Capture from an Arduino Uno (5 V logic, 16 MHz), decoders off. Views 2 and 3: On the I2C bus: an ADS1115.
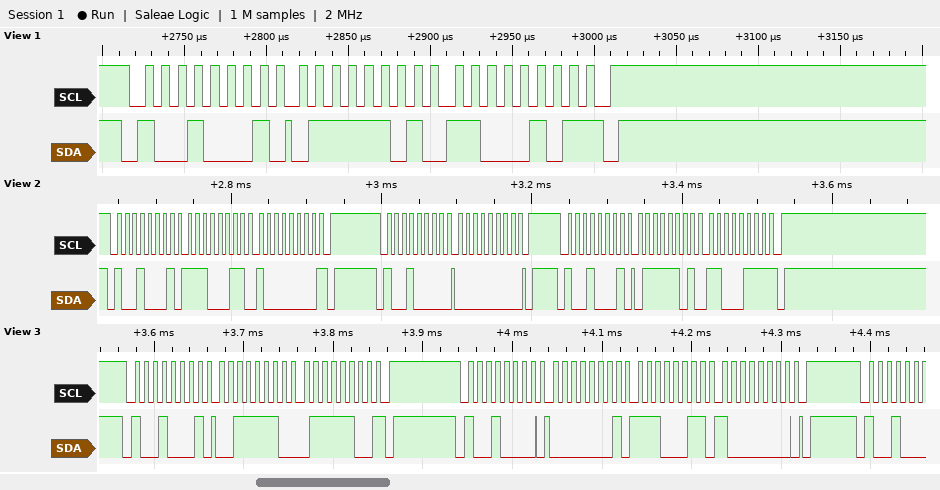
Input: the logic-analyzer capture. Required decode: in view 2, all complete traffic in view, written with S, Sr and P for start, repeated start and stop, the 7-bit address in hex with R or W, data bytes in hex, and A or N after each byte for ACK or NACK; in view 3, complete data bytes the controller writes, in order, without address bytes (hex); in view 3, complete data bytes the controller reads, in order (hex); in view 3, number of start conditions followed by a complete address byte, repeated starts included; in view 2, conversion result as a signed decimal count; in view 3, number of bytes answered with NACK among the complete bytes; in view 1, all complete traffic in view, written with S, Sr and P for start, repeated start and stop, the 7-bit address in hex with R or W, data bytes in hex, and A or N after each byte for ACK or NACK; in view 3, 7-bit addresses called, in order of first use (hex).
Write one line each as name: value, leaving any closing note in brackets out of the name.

in view 2, all complete traffic in view, written with S, Sr and P for start, repeated start and stop, the 7-bit address in hex with R or W, data bytes in hex, and A or N after each byte for ACK or NACK: S 48R A E3 A 80 N P S 48W A 00 A P S 48R A 7D A C7 N P
in view 3, complete data bytes the controller writes, in order, without address bytes: 01 E3 80
in view 3, complete data bytes the controller reads, in order: 3E 7C
in view 3, number of start conditions followed by a complete address byte, repeated starts included: 2
in view 2, conversion result as a signed decimal count: 32199
in view 3, number of bytes answered with NACK among the complete bytes: 1
in view 1, all complete traffic in view, written with S, Sr and P for start, repeated start and stop, the 7-bit address in hex with R or W, data bytes in hex, and A or N after each byte for ACK or NACK: S 48R A 7D A C5 N P
in view 3, 7-bit addresses called, in order of first use: 0x48
